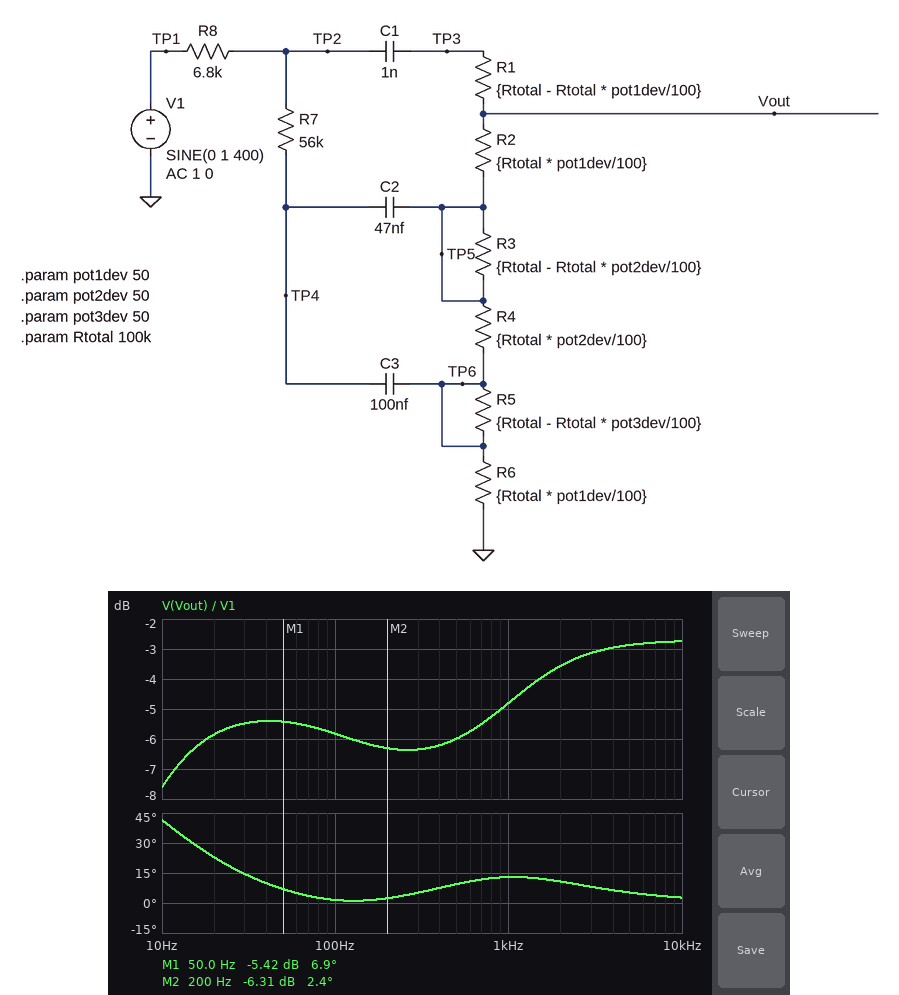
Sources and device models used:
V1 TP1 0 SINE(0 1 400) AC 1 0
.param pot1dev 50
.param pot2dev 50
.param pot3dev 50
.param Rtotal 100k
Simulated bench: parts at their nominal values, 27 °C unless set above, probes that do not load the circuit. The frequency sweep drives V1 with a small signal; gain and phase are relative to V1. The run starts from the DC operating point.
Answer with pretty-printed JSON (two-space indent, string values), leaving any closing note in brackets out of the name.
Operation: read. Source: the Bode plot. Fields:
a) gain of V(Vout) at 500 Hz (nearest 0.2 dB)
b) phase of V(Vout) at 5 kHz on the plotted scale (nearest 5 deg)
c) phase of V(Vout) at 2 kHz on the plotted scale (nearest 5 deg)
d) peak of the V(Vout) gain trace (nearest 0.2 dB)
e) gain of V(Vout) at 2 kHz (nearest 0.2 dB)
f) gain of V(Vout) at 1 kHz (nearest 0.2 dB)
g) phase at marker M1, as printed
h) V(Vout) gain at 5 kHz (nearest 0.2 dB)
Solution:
{
  "gain of V(Vout) at 500 Hz": "-6.0 dB",
  "phase of V(Vout) at 5 kHz on the plotted scale": "5 deg",
  "phase of V(Vout) at 2 kHz on the plotted scale": "10 deg",
  "peak of the V(Vout) gain trace": "-2.8 dB",
  "gain of V(Vout) at 2 kHz": "-3.6 dB",
  "gain of V(Vout) at 1 kHz": "-4.8 dB",
  "phase at marker M1, as printed": "6.9 deg",
  "V(Vout) gain at 5 kHz": "-2.8 dB"
}
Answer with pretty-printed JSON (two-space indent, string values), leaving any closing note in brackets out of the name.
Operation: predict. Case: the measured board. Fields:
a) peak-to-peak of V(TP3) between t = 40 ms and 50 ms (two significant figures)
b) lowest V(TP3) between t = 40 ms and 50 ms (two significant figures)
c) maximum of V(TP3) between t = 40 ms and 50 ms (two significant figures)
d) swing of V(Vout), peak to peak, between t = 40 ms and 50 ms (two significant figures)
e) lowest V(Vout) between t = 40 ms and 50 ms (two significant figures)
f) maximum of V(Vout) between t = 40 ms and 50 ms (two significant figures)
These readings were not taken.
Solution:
{
  "peak-to-peak of V(TP3) between t = 40 ms and 50 ms": "1.0 V",
  "lowest V(TP3) between t = 40 ms and 50 ms": "-520 mV",
  "maximum of V(TP3) between t = 40 ms and 50 ms": "510 mV",
  "swing of V(Vout), peak to peak, between t = 40 ms and 50 ms": "980 mV",
  "lowest V(Vout) between t = 40 ms and 50 ms": "-490 mV",
  "maximum of V(Vout) between t = 40 ms and 50 ms": "490 mV"
}
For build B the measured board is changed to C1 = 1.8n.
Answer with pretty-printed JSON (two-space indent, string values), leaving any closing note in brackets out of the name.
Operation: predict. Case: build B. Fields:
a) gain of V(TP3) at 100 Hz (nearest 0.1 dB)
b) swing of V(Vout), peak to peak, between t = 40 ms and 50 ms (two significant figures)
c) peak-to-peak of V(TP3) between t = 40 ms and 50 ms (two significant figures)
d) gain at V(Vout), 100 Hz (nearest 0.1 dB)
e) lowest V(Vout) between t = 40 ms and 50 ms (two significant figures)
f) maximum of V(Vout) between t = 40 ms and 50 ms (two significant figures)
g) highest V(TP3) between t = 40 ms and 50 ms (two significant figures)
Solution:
{
  "gain of V(TP3) at 100 Hz": "-5.6 dB",
  "swing of V(Vout), peak to peak, between t = 40 ms and 50 ms": "1.1 V",
  "peak-to-peak of V(TP3) between t = 40 ms and 50 ms": "1.2 V",
  "gain at V(Vout), 100 Hz": "-5.7 dB",
  "lowest V(Vout) between t = 40 ms and 50 ms": "-540 mV",
  "maximum of V(Vout) between t = 40 ms and 50 ms": "540 mV",
  "highest V(TP3) between t = 40 ms and 50 ms": "600 mV"
}
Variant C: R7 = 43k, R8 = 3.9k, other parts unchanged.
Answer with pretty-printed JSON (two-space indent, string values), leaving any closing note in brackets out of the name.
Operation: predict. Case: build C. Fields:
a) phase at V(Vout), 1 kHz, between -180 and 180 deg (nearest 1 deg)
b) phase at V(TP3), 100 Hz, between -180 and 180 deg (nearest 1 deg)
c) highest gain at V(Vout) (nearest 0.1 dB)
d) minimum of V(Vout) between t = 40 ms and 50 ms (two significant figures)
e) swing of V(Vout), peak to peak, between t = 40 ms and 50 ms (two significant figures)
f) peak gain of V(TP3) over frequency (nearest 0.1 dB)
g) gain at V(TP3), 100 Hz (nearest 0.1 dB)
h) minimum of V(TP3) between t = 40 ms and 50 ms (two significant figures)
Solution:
{
  "phase at V(Vout), 1 kHz, between -180 and 180 deg": "10 deg",
  "phase at V(TP3), 100 Hz, between -180 and 180 deg": "3 deg",
  "highest gain at V(Vout)": "-2.2 dB",
  "minimum of V(Vout) between t = 40 ms and 50 ms": "-560 mV",
  "swing of V(Vout), peak to peak, between t = 40 ms and 50 ms": "1.1 V",
  "peak gain of V(TP3) over frequency": "-0.4 dB",
  "gain at V(TP3), 100 Hz": "-4.6 dB",
  "minimum of V(TP3) between t = 40 ms and 50 ms": "-580 mV"
}
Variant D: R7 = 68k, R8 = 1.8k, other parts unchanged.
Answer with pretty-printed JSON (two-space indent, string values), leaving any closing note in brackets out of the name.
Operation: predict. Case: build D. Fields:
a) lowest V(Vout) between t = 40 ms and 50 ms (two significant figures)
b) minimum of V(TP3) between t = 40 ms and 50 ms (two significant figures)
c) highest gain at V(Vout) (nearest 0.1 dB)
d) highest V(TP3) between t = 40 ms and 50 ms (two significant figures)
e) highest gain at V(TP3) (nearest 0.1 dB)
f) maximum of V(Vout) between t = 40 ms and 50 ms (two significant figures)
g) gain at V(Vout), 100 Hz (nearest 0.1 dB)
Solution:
{
  "lowest V(Vout) between t = 40 ms and 50 ms": "-470 mV",
  "minimum of V(TP3) between t = 40 ms and 50 ms": "-510 mV",
  "highest gain at V(Vout)": "-2.4 dB",
  "highest V(TP3) between t = 40 ms and 50 ms": "500 mV",
  "highest gain at V(TP3)": "-0.2 dB",
  "maximum of V(Vout) between t = 40 ms and 50 ms": "470 mV",
  "gain at V(Vout), 100 Hz": "-6.3 dB"
}
